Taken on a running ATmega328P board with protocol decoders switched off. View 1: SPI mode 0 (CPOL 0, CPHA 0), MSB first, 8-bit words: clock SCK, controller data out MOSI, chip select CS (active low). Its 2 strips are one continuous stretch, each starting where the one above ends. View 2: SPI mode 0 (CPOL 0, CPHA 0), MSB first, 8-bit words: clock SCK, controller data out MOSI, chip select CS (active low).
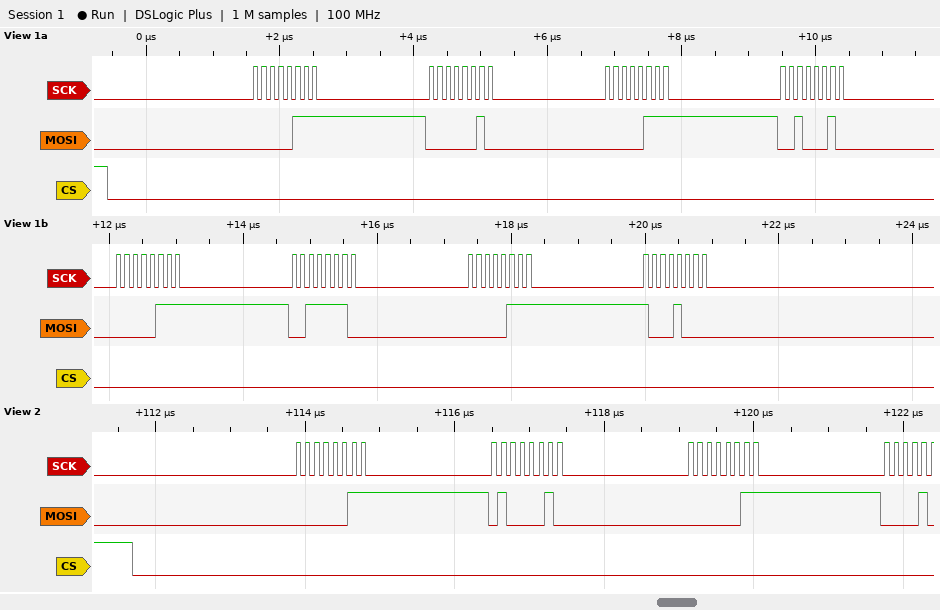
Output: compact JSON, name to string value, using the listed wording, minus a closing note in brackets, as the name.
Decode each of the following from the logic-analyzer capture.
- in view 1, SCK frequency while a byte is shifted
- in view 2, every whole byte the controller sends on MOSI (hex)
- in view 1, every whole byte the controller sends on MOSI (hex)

{"in view 1, SCK frequency while a byte is shifted": "8 MHz", "in view 2, every whole byte the controller sends on MOSI": "03 42 03", "in view 1, every whole byte the controller sends on MOSI": "07 02 07 22 07 3E 07 88"}
